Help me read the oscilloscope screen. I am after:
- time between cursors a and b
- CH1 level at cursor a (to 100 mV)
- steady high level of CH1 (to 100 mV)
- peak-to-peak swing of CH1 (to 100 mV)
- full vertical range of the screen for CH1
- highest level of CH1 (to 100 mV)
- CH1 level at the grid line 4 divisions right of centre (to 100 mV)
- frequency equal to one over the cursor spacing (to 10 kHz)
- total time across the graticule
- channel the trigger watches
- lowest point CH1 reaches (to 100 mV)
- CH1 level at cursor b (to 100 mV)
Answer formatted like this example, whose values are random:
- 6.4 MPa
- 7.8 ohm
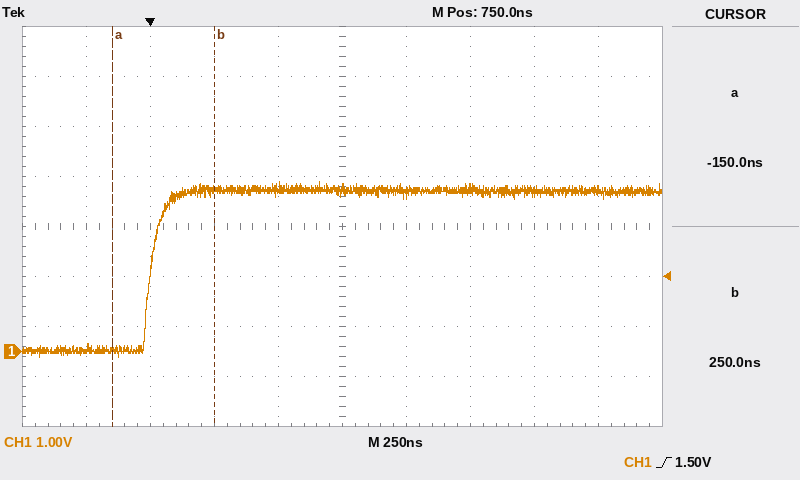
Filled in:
- 400 ns
- 0.0 V
- 3.2 V
- 3.5 V
- 8 V
- 3.4 V
- 3.2 V
- 2.50 MHz
- 2.5 µs
- CH1
- -100 mV
- 3.2 V
